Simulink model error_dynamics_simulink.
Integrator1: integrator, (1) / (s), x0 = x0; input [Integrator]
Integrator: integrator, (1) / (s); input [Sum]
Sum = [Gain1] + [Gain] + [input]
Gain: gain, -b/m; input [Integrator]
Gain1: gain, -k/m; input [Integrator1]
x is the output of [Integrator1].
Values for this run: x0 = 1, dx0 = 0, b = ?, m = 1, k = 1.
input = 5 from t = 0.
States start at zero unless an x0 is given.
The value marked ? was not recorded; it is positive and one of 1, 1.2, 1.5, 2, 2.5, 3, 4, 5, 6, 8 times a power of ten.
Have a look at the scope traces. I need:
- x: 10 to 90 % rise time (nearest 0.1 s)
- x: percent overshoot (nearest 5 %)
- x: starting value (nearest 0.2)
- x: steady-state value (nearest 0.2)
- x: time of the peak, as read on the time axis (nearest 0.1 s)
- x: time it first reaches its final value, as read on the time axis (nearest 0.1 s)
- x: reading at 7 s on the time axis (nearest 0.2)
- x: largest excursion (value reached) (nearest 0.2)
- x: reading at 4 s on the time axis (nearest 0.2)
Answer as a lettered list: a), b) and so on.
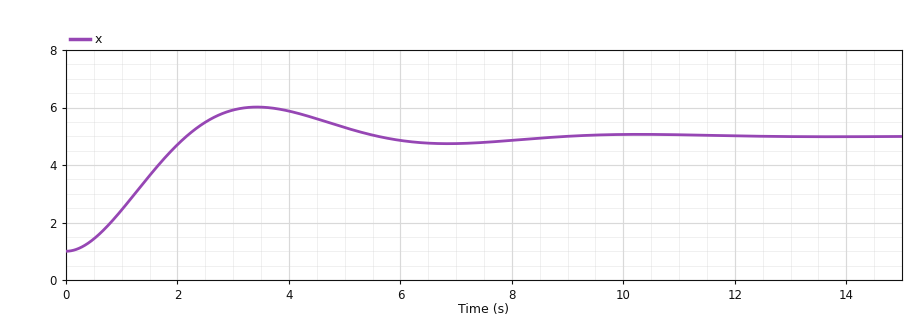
a) 1.5 s
b) 25 %
c) 1.0
d) 5.0
e) 3.4 s
f) 2.2 s
g) 4.8
h) 6.0
i) 5.8
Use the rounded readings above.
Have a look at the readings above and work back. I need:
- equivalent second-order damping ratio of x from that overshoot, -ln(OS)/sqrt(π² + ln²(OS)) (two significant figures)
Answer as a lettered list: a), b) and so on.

a) 0.40
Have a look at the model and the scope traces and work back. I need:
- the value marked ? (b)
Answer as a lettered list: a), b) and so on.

a) 0.8
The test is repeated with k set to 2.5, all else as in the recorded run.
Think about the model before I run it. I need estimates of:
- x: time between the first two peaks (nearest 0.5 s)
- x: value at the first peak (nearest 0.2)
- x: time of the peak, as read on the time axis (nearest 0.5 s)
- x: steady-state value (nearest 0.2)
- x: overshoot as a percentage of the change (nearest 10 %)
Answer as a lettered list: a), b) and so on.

a) 4.0 s
b) 2.4
c) 2.0 s
d) 2.0
e) 40 %
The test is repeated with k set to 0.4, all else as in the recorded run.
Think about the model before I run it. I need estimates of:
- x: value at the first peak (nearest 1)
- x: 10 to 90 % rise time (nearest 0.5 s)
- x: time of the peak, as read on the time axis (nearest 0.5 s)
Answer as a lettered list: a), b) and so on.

a) 13
b) 3.0 s
c) 6.5 s
